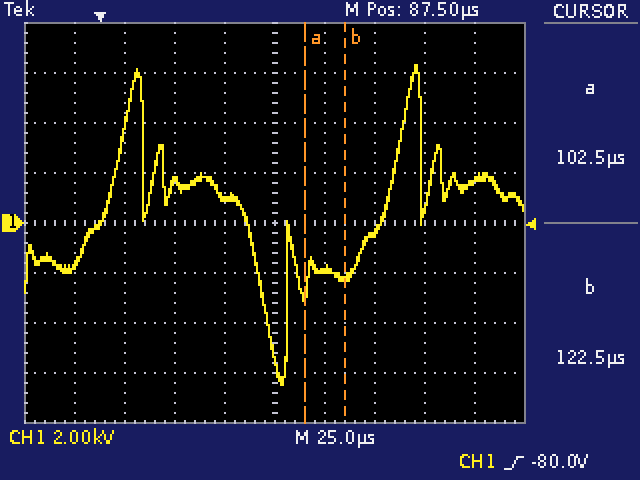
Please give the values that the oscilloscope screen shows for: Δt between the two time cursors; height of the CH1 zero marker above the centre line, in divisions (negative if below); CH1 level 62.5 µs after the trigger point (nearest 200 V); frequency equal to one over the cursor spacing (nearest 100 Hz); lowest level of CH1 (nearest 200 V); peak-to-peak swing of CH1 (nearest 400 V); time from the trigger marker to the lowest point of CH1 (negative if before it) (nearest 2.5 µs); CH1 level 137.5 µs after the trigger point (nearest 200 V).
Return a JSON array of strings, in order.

["20.0 µs", "0.0 div", "1.0 kV", "50.0 kHz", "-6.4 kV", "12.8 kV", "+90.0 µs", "-400 V"]
